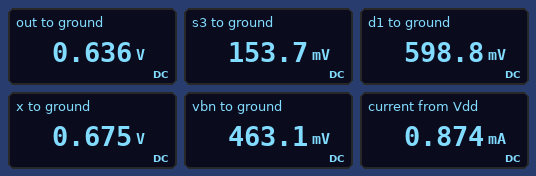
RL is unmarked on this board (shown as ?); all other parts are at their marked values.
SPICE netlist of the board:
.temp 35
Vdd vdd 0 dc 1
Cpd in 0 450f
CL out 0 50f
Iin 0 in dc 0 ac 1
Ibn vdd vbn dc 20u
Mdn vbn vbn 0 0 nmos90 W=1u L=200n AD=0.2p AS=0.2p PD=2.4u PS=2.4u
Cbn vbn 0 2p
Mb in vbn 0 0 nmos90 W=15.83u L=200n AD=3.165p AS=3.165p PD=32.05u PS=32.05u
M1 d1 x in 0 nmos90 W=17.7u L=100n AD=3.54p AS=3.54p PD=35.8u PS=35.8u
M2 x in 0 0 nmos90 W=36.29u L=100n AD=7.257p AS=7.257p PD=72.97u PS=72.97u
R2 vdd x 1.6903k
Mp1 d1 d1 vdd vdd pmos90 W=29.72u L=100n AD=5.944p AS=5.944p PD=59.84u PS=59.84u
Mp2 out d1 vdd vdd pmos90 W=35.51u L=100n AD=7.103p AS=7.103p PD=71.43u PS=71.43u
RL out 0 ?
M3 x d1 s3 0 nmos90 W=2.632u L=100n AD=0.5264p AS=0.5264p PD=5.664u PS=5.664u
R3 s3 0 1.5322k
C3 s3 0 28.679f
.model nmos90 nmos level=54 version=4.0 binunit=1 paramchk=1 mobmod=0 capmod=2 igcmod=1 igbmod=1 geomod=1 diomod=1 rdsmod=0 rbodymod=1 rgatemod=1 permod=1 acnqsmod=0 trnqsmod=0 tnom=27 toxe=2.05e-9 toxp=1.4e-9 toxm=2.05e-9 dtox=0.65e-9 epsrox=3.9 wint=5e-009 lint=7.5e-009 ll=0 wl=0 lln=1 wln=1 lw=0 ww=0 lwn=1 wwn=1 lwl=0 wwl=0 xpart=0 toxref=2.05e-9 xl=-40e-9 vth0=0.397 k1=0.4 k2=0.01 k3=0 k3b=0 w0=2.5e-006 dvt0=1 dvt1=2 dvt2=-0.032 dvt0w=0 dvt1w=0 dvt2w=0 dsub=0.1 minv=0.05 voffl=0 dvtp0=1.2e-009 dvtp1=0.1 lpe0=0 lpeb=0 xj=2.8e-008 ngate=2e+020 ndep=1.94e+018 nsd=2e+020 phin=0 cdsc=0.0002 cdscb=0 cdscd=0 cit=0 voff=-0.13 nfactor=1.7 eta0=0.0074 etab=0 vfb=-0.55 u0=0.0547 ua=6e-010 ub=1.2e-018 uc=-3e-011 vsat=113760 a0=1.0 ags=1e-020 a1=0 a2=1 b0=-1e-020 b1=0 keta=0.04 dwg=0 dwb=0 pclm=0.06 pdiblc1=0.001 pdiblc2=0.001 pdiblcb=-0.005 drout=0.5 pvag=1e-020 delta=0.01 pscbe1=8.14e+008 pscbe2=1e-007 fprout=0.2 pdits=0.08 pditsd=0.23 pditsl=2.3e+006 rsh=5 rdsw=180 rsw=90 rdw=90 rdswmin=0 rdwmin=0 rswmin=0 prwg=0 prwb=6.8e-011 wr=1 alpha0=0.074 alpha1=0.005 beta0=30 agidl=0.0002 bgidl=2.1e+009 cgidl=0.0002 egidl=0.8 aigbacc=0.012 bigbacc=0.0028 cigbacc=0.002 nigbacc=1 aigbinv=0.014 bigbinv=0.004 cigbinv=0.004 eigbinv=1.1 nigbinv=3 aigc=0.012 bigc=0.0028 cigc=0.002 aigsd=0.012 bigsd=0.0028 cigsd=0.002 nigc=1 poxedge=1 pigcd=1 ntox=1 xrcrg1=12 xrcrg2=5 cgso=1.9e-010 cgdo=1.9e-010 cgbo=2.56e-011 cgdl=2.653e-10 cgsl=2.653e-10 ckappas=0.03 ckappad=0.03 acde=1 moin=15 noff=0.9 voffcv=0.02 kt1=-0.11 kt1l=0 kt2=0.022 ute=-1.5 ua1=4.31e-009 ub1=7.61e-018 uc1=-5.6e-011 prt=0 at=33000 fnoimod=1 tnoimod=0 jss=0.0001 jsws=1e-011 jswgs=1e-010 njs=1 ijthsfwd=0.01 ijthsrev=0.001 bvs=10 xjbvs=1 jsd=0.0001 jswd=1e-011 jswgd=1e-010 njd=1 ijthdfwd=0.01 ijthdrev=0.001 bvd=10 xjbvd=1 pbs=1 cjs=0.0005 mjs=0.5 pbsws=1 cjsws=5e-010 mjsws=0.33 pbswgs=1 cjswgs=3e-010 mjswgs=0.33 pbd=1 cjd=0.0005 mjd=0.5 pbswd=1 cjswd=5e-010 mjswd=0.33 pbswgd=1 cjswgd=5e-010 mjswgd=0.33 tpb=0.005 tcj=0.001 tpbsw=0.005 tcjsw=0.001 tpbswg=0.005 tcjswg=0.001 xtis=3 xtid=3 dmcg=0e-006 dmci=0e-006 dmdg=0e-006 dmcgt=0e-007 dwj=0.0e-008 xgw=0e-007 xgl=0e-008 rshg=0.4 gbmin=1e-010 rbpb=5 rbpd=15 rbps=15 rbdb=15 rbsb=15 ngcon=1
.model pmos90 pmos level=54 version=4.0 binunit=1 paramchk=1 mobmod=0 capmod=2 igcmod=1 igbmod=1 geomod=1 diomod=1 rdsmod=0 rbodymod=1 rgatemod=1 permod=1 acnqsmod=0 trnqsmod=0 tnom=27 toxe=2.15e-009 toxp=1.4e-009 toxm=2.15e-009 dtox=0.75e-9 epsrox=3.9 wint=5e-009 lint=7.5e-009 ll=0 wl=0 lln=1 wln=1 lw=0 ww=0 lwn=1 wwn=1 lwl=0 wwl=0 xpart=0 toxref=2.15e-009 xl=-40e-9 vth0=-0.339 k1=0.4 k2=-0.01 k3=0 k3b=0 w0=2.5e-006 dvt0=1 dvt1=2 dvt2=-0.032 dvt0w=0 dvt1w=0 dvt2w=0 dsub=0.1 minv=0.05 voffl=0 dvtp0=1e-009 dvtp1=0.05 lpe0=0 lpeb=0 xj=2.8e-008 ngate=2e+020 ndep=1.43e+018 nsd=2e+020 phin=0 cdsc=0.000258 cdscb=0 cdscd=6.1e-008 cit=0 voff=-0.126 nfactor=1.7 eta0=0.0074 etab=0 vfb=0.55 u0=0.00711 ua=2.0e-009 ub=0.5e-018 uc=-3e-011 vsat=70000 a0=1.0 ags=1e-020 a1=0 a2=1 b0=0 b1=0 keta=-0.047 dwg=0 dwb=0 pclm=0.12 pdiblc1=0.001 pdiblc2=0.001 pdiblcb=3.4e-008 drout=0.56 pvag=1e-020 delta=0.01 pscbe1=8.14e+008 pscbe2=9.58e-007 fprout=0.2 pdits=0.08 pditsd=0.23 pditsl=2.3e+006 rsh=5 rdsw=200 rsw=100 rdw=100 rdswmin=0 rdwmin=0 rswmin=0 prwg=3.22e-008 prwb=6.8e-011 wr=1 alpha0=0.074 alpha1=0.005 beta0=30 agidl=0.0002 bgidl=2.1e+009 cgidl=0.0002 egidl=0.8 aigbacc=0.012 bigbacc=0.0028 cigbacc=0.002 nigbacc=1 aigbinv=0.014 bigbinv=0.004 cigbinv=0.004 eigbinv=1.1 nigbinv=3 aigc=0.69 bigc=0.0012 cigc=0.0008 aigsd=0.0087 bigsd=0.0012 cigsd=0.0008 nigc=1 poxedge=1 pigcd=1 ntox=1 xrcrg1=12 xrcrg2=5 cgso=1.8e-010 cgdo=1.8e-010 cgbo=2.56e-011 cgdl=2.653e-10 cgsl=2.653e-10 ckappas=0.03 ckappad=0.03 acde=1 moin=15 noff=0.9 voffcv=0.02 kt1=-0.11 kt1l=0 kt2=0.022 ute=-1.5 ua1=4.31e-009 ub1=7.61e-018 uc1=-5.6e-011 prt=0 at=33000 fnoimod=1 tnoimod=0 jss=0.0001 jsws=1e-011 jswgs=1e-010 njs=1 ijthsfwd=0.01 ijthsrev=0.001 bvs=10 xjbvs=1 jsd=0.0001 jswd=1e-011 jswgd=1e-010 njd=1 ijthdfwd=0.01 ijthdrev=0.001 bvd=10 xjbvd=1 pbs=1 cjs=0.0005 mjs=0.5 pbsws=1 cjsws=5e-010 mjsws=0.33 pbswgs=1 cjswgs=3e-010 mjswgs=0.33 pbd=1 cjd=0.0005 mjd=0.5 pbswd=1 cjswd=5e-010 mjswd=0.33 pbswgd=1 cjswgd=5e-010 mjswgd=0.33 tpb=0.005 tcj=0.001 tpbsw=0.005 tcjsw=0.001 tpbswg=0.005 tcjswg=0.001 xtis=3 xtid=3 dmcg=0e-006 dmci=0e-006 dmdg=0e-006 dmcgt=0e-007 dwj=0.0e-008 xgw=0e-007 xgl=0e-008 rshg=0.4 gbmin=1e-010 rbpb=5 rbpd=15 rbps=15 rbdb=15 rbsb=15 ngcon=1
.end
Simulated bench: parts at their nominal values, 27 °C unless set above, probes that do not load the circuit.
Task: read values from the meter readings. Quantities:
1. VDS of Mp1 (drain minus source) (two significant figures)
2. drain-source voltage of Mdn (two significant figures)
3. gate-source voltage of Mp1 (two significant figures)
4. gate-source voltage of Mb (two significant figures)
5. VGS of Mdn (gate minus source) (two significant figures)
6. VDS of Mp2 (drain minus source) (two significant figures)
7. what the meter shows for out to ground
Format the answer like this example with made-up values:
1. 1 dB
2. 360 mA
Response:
1. -400 mV
2. 460 mV
3. -400 mV
4. 460 mV
5. 460 mV
6. -360 mV
7. 0.636 V
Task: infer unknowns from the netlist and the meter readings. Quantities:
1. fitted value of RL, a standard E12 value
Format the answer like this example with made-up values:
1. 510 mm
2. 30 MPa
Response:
1. 1.8 kΩ
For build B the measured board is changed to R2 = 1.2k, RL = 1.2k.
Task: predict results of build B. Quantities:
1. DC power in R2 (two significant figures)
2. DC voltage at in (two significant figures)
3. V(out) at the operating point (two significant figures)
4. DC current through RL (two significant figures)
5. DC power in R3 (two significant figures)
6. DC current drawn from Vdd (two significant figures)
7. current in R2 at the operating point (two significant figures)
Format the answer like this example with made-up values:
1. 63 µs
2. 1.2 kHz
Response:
1. 74 µW
2. 270 mV
3. 500 mV
4. 410 µA
5. 16 µW
6. 990 µA
7. 250 µA
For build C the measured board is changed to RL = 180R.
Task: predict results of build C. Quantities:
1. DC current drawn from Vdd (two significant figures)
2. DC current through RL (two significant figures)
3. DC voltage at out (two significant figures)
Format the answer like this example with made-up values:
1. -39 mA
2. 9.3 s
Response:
1. 1.1 mA
2. 600 µA
3. 110 mV
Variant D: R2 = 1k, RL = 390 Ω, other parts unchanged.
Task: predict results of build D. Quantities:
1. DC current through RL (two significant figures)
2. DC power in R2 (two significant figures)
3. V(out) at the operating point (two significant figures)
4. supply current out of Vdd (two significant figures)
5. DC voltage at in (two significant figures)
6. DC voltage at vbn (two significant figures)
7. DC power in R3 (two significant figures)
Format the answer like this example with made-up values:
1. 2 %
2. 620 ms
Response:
1. 550 µA
2. 81 µW
3. 210 mV
4. 1.2 mA
5. 280 mV
6. 460 mV
7. 16 µW
